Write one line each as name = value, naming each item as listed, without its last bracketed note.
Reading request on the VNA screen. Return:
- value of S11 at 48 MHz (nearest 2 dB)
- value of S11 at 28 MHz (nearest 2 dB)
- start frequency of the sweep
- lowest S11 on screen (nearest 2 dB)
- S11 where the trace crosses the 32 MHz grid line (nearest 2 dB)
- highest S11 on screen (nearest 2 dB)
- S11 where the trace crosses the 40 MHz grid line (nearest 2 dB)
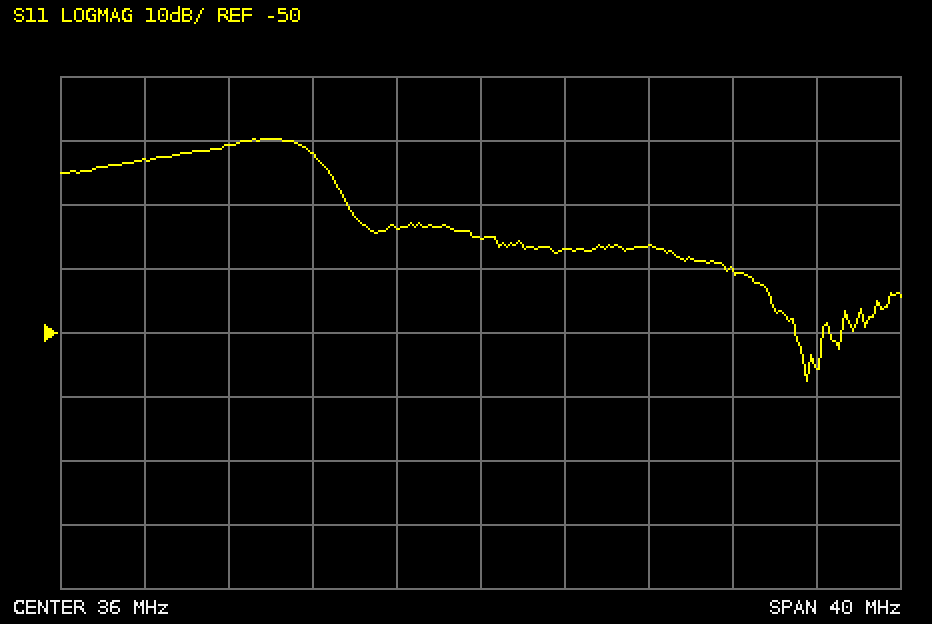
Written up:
value of S11 at 48 MHz = -40 dB
value of S11 at 28 MHz = -22 dB
start frequency of the sweep = 16 MHz
lowest S11 on screen = -58 dB
S11 where the trace crosses the 32 MHz grid line = -34 dB
highest S11 on screen = -20 dB
S11 where the trace crosses the 40 MHz grid line = -36 dB
